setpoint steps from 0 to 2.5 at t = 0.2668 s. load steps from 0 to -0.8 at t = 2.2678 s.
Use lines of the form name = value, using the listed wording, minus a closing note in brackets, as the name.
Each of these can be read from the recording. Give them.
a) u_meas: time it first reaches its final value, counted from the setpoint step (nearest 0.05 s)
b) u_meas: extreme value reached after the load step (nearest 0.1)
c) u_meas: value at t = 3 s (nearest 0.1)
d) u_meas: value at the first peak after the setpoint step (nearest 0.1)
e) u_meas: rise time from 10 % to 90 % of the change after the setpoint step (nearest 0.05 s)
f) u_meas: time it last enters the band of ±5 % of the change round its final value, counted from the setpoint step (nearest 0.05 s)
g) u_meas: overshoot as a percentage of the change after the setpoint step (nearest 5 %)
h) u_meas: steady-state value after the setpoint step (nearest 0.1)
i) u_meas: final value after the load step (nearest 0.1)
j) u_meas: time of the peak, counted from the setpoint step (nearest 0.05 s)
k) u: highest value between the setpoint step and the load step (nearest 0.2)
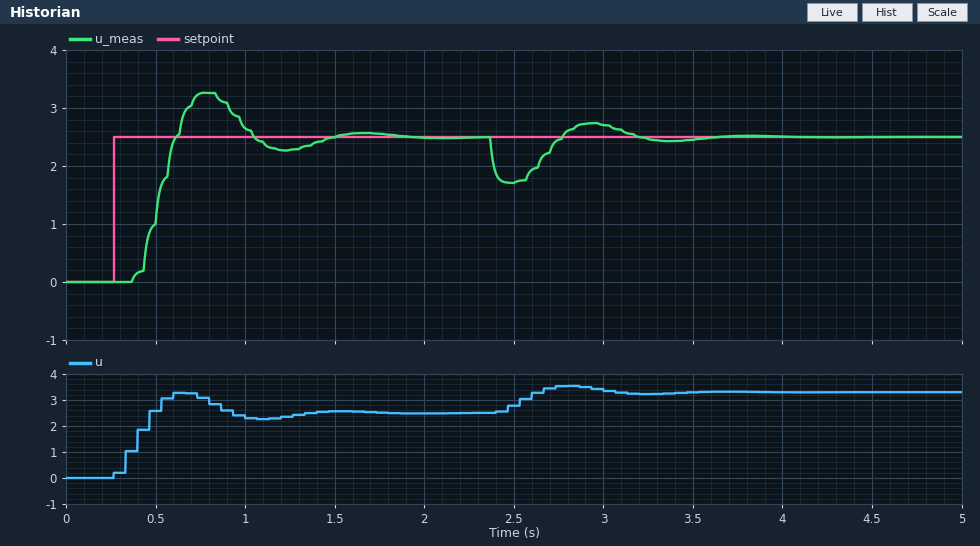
u_meas: time it first reaches its final value, counted from the setpoint step = 0.35 s
u_meas: extreme value reached after the load step = 1.7
u_meas: value at t = 3 s = 2.7
u_meas: value at the first peak after the setpoint step = 3.3
u_meas: rise time from 10 % to 90 % of the change after the setpoint step = 0.15 s
u_meas: time it last enters the band of ±5 % of the change round its final value, counted from the setpoint step = 1.10 s
u_meas: overshoot as a percentage of the change after the setpoint step = 30 %
u_meas: steady-state value after the setpoint step = 2.5
u_meas: final value after the load step = 2.5
u_meas: time of the peak, counted from the setpoint step = 0.50 s
u: highest value between the setpoint step and the load step = 3.2
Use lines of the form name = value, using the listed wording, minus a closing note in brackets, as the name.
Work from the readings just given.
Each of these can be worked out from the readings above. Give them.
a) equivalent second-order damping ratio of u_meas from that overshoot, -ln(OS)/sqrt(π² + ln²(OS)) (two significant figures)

equivalent second-order damping ratio of u_meas from that overshoot, -ln(OS)/sqrt(π² + ln²(OS)) = 0.36
